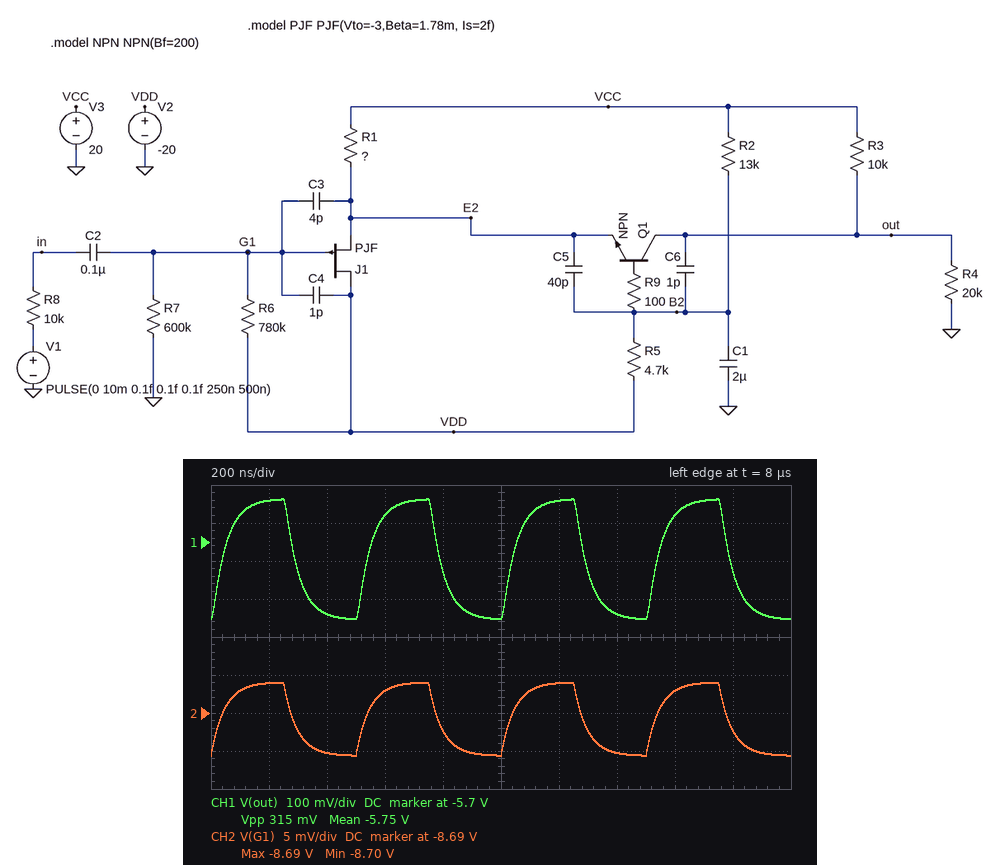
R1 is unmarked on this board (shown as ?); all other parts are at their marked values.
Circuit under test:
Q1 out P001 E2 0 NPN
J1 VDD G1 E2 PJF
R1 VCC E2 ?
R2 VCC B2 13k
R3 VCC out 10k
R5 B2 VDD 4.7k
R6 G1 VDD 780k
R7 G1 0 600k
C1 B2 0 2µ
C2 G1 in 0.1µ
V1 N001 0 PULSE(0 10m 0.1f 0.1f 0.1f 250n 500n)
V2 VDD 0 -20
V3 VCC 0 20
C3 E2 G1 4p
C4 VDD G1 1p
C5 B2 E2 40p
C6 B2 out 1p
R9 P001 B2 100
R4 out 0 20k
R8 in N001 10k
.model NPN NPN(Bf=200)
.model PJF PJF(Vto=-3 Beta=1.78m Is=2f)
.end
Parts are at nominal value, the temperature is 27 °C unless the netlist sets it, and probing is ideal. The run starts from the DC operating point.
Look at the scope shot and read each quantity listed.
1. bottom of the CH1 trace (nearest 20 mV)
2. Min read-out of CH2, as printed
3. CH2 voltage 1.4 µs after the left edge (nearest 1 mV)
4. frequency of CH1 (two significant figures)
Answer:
-5.90 V
-8.70 V
-8.695 V
2.0 MHz
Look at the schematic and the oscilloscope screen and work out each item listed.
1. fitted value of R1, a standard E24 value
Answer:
33 kΩ
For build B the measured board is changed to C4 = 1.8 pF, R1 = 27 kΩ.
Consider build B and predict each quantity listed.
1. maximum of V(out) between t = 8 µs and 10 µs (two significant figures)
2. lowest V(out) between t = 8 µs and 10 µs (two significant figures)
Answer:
-4.4 V
-4.7 V
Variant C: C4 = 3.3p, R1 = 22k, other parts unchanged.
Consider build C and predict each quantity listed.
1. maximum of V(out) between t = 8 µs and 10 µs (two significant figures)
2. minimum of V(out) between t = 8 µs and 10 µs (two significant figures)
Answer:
-2.9 V
-3.2 V
